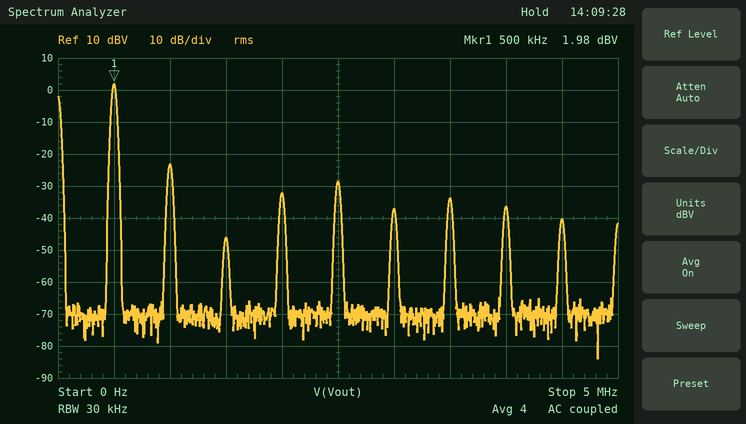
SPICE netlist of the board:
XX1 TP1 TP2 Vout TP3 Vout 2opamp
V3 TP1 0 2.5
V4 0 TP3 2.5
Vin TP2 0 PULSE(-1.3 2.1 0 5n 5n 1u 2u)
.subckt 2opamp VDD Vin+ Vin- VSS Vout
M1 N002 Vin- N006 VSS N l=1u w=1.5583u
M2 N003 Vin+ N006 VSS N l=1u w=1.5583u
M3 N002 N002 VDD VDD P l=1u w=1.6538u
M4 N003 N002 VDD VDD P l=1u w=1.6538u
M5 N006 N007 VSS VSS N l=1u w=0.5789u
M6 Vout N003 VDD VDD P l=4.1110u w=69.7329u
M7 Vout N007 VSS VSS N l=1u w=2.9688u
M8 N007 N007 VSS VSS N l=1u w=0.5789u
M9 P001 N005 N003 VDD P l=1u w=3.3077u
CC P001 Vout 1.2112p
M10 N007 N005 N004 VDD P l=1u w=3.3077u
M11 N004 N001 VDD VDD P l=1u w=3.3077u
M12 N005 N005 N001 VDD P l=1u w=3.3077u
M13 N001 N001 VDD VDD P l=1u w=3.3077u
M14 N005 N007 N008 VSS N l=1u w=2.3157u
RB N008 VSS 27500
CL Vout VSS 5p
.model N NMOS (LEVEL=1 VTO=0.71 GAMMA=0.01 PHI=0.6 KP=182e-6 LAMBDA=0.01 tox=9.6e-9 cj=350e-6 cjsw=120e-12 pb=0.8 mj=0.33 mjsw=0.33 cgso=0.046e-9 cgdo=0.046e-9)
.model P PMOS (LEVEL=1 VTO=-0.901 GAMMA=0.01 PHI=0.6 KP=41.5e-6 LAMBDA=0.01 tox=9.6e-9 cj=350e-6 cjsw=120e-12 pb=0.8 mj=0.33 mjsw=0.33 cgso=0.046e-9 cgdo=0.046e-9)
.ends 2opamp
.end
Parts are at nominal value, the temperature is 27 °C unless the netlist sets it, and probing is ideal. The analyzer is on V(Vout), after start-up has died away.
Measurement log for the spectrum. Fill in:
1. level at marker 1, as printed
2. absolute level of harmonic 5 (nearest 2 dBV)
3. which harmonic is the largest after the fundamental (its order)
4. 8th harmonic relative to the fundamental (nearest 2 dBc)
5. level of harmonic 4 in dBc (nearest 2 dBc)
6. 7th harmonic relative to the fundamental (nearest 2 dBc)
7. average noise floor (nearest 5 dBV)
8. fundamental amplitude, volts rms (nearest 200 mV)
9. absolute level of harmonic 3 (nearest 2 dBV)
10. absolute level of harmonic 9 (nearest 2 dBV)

1.98 dBV
-28 dBV
2
-38 dBc
-34 dBc
-36 dBc
-70 dBV
1.2 V
-46 dBV
-40 dBV
